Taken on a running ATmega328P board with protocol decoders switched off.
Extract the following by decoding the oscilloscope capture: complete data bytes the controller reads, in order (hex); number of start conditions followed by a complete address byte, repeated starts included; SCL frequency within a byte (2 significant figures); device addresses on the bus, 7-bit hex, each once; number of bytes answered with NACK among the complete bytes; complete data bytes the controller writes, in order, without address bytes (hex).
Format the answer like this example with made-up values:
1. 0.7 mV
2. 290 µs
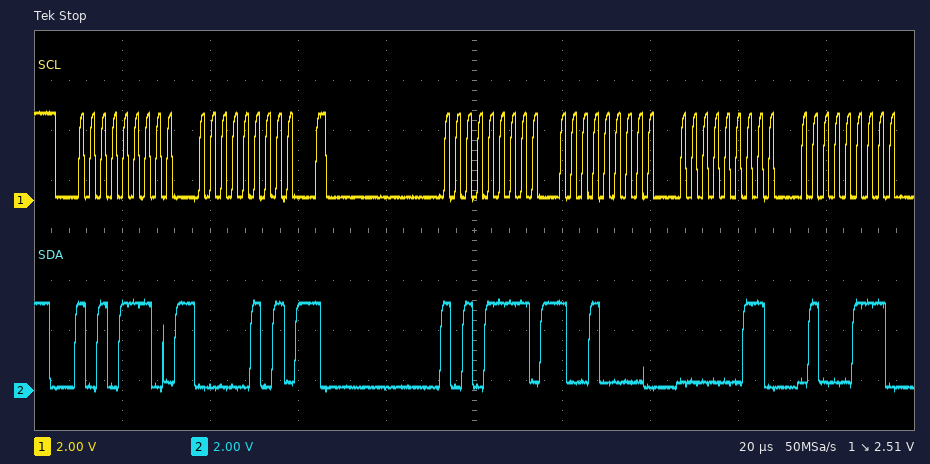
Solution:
1. 90 03 47
2. 2
3. 400 kHz
4. 0x57
5. 0
6. 05
